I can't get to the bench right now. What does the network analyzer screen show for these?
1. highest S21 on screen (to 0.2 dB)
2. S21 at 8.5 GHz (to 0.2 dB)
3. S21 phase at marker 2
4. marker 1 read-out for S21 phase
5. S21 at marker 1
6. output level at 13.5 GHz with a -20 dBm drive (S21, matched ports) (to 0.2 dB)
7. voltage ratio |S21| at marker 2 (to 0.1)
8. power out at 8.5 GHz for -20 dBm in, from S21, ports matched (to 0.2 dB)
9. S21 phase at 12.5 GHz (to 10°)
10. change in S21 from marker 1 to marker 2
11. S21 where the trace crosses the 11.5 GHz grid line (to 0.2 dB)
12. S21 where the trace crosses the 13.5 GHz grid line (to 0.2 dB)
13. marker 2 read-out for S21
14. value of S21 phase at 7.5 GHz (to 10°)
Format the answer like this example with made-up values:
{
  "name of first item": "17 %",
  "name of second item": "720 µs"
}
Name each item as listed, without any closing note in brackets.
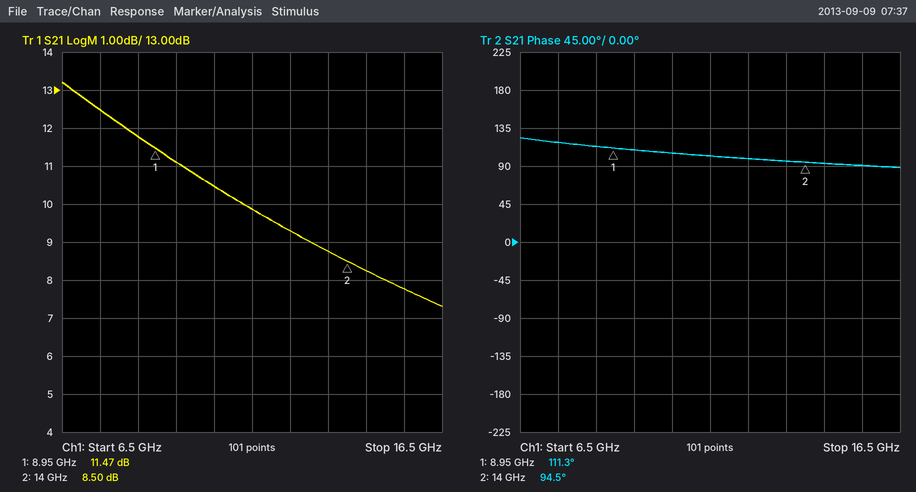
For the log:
{
  "highest S21 on screen": "13.2 dB",
  "S21 at 8.5 GHz": "11.8 dB",
  "S21 phase at marker 2": "94.5°",
  "marker 1 read-out for S21 phase": "111.3°",
  "S21 at marker 1": "11.47 dB",
  "output level at 13.5 GHz with a -20 dBm drive (S21, matched ports)": "-11.2 dBm",
  "voltage ratio |S21| at marker 2": "2.7",
  "power out at 8.5 GHz for -20 dBm in, from S21, ports matched": "-8.2 dBm",
  "S21 phase at 12.5 GHz": "100°",
  "change in S21 from marker 1 to marker 2": "-2.97 dB",
  "S21 where the trace crosses the 11.5 GHz grid line": "9.8 dB",
  "S21 where the trace crosses the 13.5 GHz grid line": "8.8 dB",
  "marker 2 read-out for S21": "8.50 dB",
  "value of S21 phase at 7.5 GHz": "120°"
}
